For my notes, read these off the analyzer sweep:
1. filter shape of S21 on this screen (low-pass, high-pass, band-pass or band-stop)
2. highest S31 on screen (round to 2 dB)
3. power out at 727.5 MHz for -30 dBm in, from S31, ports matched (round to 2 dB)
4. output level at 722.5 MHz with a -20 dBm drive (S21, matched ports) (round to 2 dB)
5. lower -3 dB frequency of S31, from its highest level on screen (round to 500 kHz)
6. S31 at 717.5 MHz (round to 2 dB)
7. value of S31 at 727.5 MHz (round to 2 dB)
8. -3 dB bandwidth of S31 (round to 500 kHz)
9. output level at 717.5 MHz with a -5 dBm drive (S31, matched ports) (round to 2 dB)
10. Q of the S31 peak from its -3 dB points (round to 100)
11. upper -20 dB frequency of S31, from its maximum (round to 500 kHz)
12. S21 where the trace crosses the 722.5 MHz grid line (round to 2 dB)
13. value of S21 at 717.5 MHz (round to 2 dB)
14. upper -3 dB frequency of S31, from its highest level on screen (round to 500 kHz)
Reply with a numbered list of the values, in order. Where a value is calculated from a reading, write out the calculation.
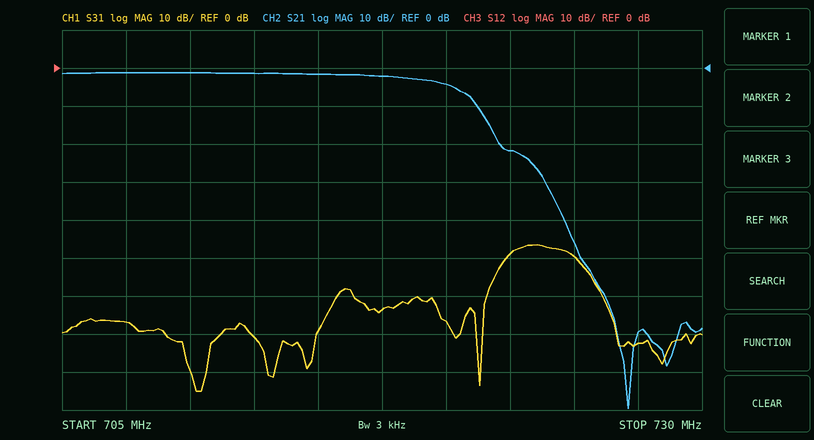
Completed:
1. low-pass
2. -46 dB
3. -30 dBm + (-72 dB) = -102 dBm
4. -20 dBm + (-22 dB) = -42 dBm
5. 722.5 MHz
6. -64 dB
7. -72 dB
8. 725.0 MHz − 722.5 MHz = 2.5 MHz
9. -5 dBm + (-64 dB) = -68 dBm
10. 723.75 MHz / 2.5 MHz ≈ 290, so 300 to the nearest 100
11. 726.5 MHz
12. -22 dB
13. -2 dB
14. 725.0 MHz
